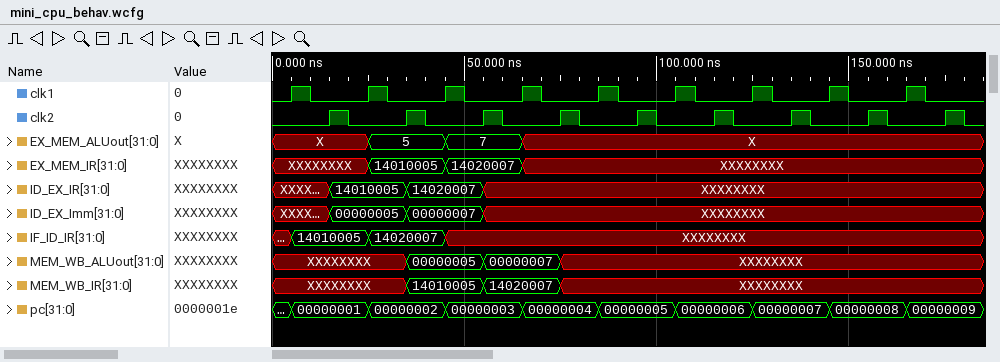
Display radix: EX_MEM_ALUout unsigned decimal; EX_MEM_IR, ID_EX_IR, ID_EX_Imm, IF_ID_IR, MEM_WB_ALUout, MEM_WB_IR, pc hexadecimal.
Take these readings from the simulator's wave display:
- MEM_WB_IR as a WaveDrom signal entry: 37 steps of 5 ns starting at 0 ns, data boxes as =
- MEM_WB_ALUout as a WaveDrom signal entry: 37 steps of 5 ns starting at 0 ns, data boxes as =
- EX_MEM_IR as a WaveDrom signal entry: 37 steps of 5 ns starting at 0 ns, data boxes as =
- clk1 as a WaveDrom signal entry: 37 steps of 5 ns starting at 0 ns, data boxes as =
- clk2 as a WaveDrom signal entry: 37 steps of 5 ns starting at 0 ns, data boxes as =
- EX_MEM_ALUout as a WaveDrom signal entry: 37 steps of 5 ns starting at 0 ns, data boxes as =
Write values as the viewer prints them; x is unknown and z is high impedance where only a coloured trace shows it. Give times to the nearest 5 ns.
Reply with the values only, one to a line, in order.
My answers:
{name: 'MEM_WB_IR', wave: 'x......=...=...x.....................', data: '14010005 14020007'}
{name: 'MEM_WB_ALUout', wave: 'x......=...=...x.....................', data: '00000005 00000007'}
{name: 'EX_MEM_IR', wave: 'x....=...=...x.......................', data: '14010005 14020007'}
{name: 'clk1', wave: '010..10..10..10..10..10..10..10..10..'}
{name: 'clk2', wave: '0..10..10..10..10..10..10..10..10..10'}
{name: 'EX_MEM_ALUout', wave: 'x....=...=...x.......................', data: '5 7'}
